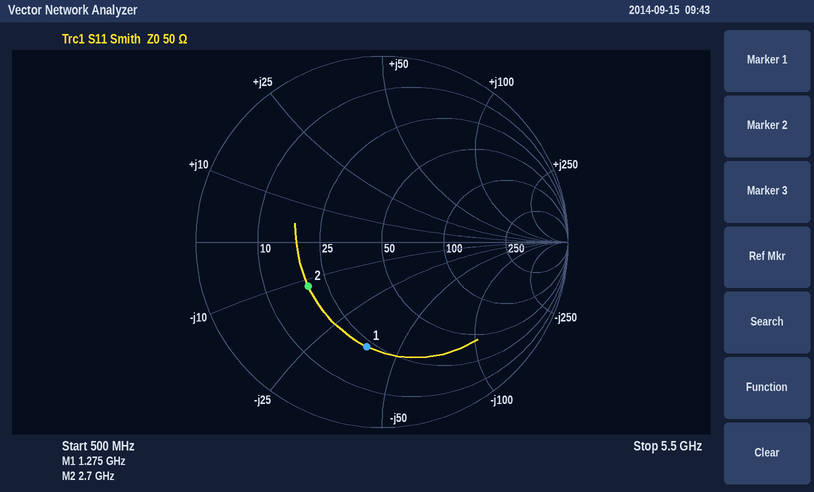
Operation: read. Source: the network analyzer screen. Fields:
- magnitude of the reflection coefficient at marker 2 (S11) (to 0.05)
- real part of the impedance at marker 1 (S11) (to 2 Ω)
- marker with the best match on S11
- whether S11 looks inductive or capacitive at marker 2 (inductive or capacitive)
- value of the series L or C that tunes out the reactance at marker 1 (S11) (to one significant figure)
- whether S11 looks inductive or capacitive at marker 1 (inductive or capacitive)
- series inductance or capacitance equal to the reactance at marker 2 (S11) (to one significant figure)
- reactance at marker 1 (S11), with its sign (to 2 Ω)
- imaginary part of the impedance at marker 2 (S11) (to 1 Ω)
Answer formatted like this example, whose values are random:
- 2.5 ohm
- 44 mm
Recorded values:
- 0.45
- 22 Ω
- marker 2
- capacitive
- 5 nH
- capacitive
- 5 pF
- -38 Ω
- -12 Ω
